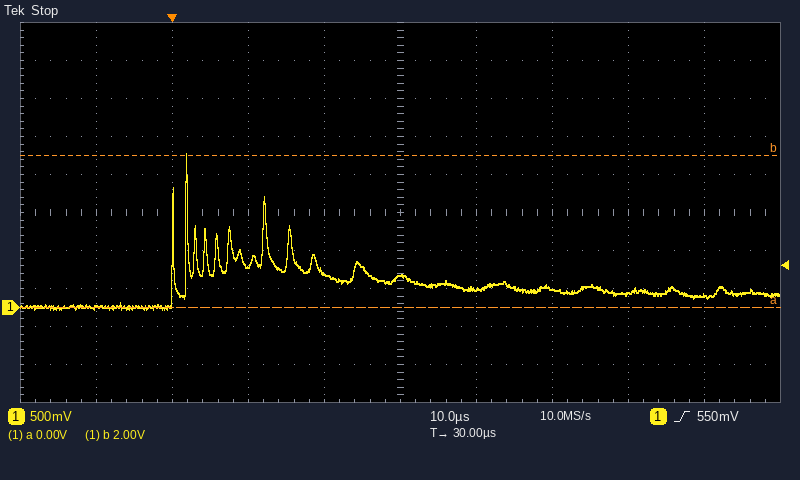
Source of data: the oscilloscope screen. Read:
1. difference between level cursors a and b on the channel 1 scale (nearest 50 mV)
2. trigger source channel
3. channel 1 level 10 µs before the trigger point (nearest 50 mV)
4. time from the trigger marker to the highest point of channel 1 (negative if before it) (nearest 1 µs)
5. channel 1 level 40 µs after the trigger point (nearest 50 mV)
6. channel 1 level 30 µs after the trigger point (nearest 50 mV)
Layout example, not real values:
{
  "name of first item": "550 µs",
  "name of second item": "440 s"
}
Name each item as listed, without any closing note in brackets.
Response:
{
  "difference between level cursors a and b on the channel 1 scale": "2.00 V",
  "trigger source channel": "channel 1",
  "channel 1 level 10 µs before the trigger point": "0 mV",
  "time from the trigger marker to the highest point of channel 1 (negative if before it)": "+2 µs",
  "channel 1 level 40 µs after the trigger point": "250 mV",
  "channel 1 level 30 µs after the trigger point": "400 mV"
}
